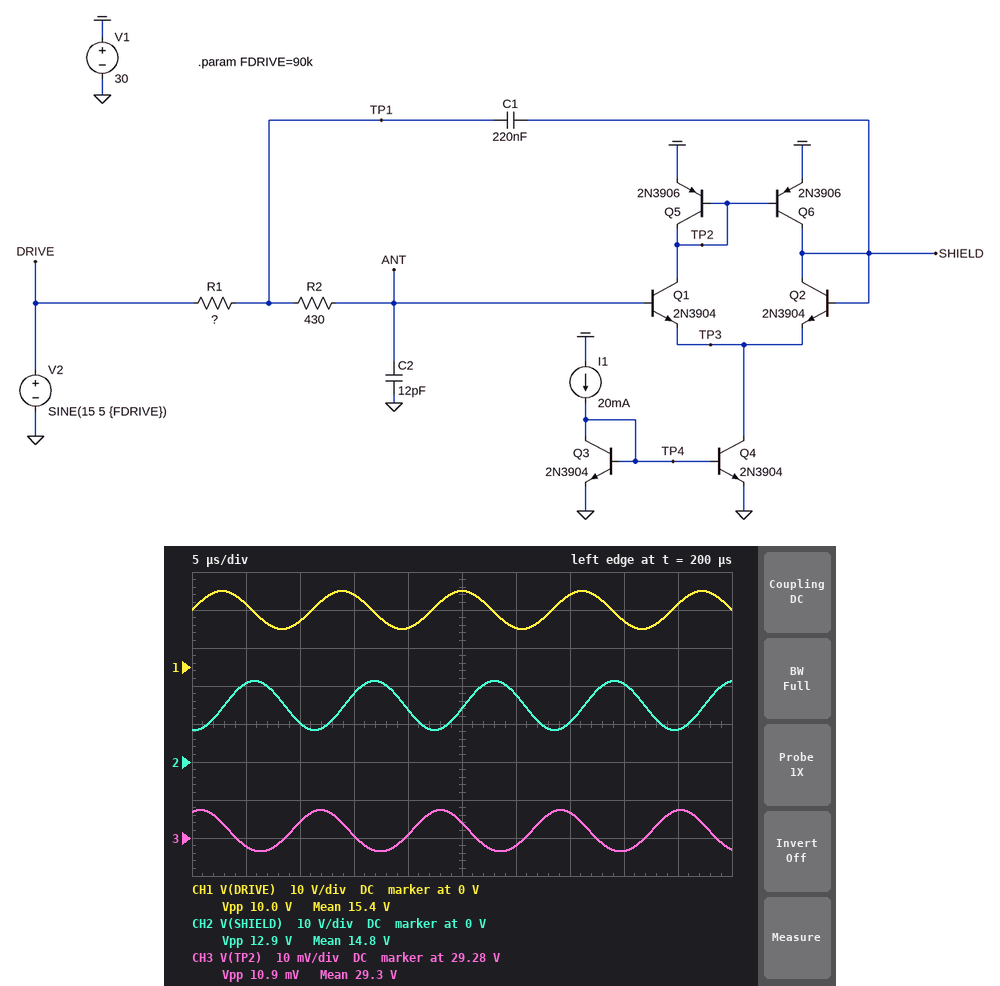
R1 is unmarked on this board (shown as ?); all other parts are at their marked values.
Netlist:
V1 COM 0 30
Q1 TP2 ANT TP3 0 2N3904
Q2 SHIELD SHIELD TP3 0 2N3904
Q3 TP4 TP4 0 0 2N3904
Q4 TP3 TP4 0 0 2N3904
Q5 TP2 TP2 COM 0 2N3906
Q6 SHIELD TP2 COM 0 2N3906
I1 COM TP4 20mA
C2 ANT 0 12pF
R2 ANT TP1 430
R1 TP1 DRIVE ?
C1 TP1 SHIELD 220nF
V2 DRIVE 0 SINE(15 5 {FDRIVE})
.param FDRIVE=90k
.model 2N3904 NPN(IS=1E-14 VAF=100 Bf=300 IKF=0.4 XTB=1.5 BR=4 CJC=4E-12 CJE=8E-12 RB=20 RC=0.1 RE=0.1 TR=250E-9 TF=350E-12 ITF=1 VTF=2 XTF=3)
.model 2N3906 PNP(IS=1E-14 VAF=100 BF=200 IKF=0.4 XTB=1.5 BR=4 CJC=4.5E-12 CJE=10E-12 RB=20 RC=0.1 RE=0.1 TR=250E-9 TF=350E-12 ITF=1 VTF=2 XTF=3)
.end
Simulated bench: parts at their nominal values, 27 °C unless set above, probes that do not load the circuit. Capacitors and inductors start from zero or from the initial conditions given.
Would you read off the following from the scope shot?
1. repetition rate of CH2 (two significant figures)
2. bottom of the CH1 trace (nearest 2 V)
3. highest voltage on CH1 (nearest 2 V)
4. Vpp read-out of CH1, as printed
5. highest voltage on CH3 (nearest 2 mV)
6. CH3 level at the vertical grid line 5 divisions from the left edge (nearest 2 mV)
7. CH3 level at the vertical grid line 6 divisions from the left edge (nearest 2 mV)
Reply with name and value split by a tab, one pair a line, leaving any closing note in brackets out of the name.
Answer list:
repetition rate of CH2	90 kHz
bottom of the CH1 trace	10 V
highest voltage on CH1	20 V
Vpp read-out of CH1, as printed	10.0 V
highest voltage on CH3	29.288 V
CH3 level at the vertical grid line 5 divisions from the left edge	29.284 V
CH3 level at the vertical grid line 6 divisions from the left edge	29.278 V
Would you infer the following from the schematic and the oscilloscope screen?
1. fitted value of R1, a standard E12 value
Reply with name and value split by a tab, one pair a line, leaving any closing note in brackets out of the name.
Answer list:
fitted value of R1, a standard E12 value	3.3 kΩ
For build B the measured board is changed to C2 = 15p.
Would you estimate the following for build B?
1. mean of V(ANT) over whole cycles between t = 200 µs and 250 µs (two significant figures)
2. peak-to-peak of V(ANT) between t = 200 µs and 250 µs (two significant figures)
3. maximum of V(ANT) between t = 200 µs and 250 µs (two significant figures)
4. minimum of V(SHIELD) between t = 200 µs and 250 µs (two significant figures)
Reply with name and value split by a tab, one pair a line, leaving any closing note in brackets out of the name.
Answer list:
mean of V(ANT) over whole cycles between t = 200 µs and 250 µs	15 V
peak-to-peak of V(ANT) between t = 200 µs and 250 µs	11 V
maximum of V(ANT) between t = 200 µs and 250 µs	20 V
minimum of V(SHIELD) between t = 200 µs and 250 µs	9.6 V
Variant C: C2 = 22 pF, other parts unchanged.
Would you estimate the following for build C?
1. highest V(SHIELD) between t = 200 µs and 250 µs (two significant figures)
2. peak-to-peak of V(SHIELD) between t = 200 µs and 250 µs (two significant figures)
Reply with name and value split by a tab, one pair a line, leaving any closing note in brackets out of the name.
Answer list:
highest V(SHIELD) between t = 200 µs and 250 µs	18 V
peak-to-peak of V(SHIELD) between t = 200 µs and 250 µs	6.7 V
